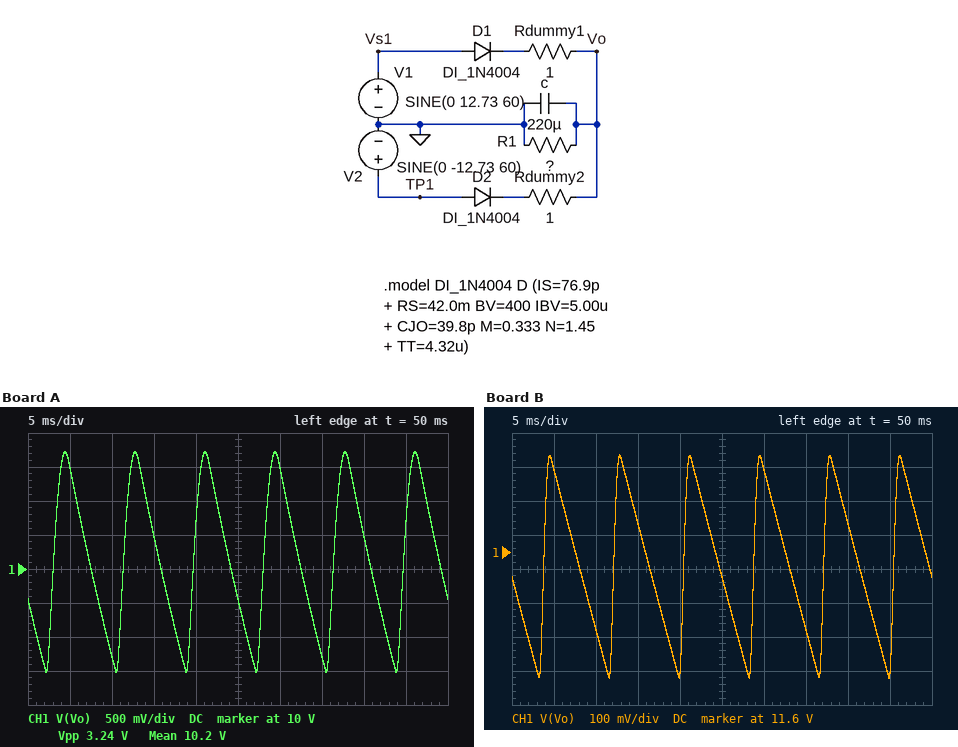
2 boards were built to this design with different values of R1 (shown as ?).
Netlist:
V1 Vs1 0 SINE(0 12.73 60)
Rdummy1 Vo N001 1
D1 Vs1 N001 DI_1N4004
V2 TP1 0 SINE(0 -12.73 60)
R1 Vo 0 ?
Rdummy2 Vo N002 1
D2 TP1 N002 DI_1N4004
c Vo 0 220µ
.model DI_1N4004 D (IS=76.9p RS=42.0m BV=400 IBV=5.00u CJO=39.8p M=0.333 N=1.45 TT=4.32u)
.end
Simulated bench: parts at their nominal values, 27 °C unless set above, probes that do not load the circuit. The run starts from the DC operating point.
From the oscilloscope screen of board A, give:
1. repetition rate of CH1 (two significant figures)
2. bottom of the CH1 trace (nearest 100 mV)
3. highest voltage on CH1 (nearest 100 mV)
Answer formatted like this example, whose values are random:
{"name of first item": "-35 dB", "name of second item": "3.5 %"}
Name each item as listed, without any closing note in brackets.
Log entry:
{"repetition rate of CH1": "120 Hz", "bottom of the CH1 trace": "8.5 V", "highest voltage on CH1": "11.7 V"}
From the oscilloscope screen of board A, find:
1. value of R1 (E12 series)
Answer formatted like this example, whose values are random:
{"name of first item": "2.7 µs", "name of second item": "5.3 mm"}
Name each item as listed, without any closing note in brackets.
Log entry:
{"value of R1": "82 Ω"}
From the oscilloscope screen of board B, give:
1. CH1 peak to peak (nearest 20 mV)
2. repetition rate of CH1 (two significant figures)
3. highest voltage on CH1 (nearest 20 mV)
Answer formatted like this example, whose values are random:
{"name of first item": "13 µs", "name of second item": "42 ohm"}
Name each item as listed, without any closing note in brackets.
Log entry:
{"CH1 peak to peak": "660 mV", "repetition rate of CH1": "120 Hz", "highest voltage on CH1": "11.88 V"}
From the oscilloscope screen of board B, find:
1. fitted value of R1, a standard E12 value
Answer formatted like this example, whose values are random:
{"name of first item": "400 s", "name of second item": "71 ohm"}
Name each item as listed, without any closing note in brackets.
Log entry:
{"fitted value of R1, a standard E12 value": "560 Ω"}
